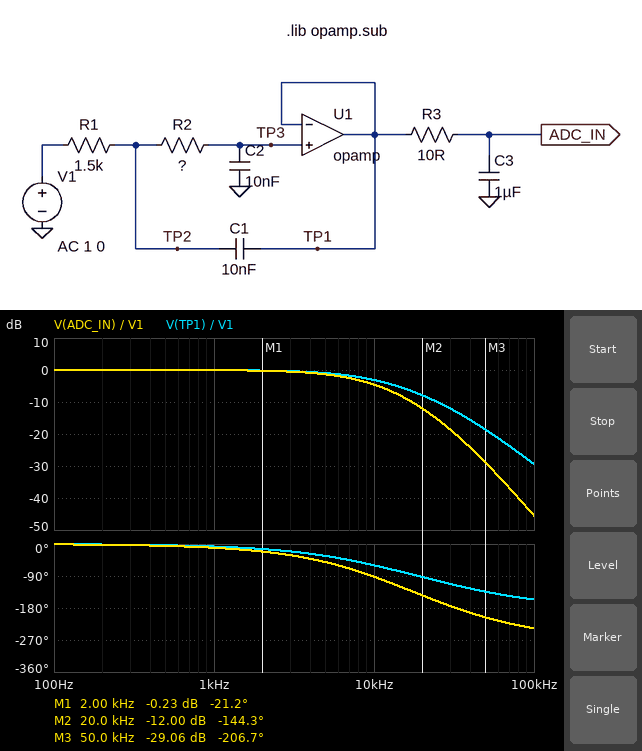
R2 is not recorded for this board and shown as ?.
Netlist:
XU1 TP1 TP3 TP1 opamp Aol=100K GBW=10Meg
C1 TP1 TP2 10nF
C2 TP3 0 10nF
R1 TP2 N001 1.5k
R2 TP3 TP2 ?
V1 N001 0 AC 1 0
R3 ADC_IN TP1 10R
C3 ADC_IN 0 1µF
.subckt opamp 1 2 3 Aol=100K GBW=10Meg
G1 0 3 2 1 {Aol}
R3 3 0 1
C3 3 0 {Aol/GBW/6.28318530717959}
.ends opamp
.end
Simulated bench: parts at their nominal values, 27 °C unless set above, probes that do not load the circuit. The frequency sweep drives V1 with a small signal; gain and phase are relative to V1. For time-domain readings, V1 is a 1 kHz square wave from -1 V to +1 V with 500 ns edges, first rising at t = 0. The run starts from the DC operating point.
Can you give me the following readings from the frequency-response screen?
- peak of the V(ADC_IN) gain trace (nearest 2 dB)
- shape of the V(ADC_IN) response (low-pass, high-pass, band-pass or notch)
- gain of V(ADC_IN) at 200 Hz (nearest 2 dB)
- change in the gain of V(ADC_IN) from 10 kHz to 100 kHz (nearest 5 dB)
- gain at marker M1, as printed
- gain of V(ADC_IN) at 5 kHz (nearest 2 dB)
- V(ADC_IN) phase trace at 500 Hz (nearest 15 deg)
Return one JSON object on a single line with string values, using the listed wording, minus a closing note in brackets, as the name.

{"peak of the V(ADC_IN) gain trace": "0 dB", "shape of the V(ADC_IN) response": "low-pass", "gain of V(ADC_IN) at 200 Hz": "0 dB", "change in the gain of V(ADC_IN) from 10 kHz to 100 kHz": "-40 dB", "gain at marker M1, as printed": "-0.23 dB", "gain of V(ADC_IN) at 5 kHz": "-2 dB", "V(ADC_IN) phase trace at 500 Hz": "0 deg"}
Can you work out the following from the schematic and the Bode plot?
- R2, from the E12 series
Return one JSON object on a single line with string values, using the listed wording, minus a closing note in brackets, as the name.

{"R2, from the E12 series": "470 Ω"}
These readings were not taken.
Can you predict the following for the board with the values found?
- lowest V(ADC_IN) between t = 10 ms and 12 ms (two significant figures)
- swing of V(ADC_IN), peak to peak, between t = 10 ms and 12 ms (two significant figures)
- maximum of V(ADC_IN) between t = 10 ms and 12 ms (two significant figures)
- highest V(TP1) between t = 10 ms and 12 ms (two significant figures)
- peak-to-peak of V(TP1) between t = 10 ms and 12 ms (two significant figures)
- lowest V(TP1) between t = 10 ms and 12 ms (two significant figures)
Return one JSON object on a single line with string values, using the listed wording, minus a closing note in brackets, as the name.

{"lowest V(ADC_IN) between t = 10 ms and 12 ms": "-1.0 V", "swing of V(ADC_IN), peak to peak, between t = 10 ms and 12 ms": "2.0 V", "maximum of V(ADC_IN) between t = 10 ms and 12 ms": "1.0 V", "highest V(TP1) between t = 10 ms and 12 ms": "1.0 V", "peak-to-peak of V(TP1) between t = 10 ms and 12 ms": "2.0 V", "lowest V(TP1) between t = 10 ms and 12 ms": "-1.0 V"}
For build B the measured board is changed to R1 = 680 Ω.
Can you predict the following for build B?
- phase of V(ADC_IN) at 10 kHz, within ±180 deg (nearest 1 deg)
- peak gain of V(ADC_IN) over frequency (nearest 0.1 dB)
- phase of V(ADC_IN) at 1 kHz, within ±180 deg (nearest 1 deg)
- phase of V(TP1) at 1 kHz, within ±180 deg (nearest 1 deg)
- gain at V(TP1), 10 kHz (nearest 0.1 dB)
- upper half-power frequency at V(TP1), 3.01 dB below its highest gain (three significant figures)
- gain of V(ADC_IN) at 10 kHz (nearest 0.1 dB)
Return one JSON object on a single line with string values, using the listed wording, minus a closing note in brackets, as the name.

{"phase of V(ADC_IN) at 10 kHz, within ±180 deg": "-72 deg", "peak gain of V(ADC_IN) over frequency": "0 dB", "phase of V(ADC_IN) at 1 kHz, within ±180 deg": "-8 deg", "phase of V(TP1) at 1 kHz, within ±180 deg": "-4 deg", "gain at V(TP1), 10 kHz": "-1.1 dB", "upper half-power frequency at V(TP1), 3.01 dB below its highest gain": "17.7 kHz", "gain of V(ADC_IN) at 10 kHz": "-2.5 dB"}
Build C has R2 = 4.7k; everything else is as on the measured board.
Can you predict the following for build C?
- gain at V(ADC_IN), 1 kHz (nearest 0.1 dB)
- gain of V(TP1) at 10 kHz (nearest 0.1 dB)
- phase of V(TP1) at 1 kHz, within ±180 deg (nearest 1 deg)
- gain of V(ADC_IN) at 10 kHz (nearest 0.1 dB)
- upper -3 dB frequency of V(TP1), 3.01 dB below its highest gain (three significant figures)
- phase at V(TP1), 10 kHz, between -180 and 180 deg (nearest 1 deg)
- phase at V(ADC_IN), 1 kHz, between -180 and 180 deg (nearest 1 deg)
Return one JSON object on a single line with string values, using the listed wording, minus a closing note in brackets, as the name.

{"gain at V(ADC_IN), 1 kHz": "-0.4 dB", "gain of V(TP1) at 10 kHz": "-12.6 dB", "phase of V(TP1) at 1 kHz, within ±180 deg": "-22 deg", "gain of V(ADC_IN) at 10 kHz": "-14.1 dB", "upper -3 dB frequency of V(TP1), 3.01 dB below its highest gain": "3.11 kHz", "phase at V(TP1), 10 kHz, between -180 and 180 deg": "-115 deg", "phase at V(ADC_IN), 1 kHz, between -180 and 180 deg": "-25 deg"}
